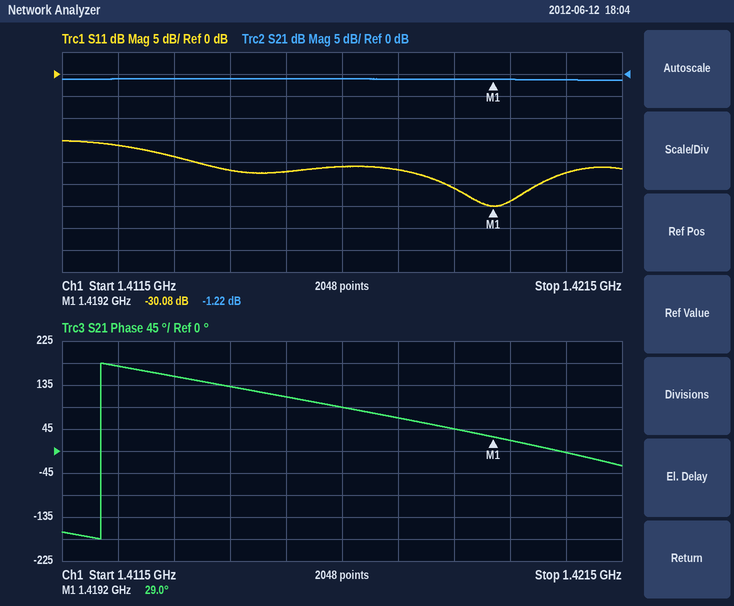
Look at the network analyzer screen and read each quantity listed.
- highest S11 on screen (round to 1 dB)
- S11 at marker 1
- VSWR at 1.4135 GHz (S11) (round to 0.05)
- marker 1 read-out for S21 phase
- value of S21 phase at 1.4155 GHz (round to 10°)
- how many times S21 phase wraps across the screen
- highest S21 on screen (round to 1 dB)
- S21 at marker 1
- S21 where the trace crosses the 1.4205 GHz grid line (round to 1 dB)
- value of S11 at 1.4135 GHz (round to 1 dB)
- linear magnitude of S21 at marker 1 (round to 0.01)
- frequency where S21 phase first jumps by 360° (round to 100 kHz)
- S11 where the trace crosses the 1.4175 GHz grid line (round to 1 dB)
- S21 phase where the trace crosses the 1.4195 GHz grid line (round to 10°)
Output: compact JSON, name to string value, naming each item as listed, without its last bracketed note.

{"highest S11 on screen": "-15 dB", "S11 at marker 1": "-30.08 dB", "VSWR at 1.4135 GHz (S11)": "1.25", "marker 1 read-out for S21 phase": "29.0°", "value of S21 phase at 1.4155 GHz": "110°", "how many times S21 phase wraps across the screen": "1", "highest S21 on screen": "-1 dB", "S21 at marker 1": "-1.22 dB", "S21 where the trace crosses the 1.4205 GHz grid line": "-1 dB", "value of S11 at 1.4135 GHz": "-19 dB", "linear magnitude of S21 at marker 1": "0.87", "frequency where S21 phase first jumps by 360°": "1.4122 GHz", "S11 where the trace crosses the 1.4175 GHz grid line": "-22 dB", "S21 phase where the trace crosses the 1.4195 GHz grid line": "20°"}
